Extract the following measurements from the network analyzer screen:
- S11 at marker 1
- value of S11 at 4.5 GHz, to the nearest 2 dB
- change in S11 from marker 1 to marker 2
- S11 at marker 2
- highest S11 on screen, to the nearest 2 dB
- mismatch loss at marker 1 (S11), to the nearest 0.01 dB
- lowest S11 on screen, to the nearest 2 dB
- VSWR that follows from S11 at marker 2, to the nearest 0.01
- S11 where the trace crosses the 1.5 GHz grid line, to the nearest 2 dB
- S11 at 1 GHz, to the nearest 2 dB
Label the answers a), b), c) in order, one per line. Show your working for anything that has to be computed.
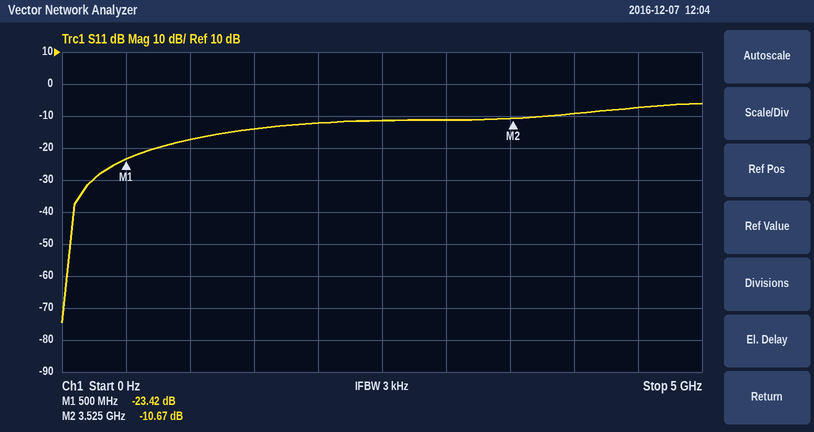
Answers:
a) -23.42 dB
b) -8 dB
c) -10.67 − (-23.42) = 12.75 dB
d) -10.67 dB
e) -6 dB
f) −10 log10(1 − 10^(-23.42/10)) ≈ 0.02 dB
g) -74 dB
h) (1 + 0.2928)/(1 − 0.2928) ≈ 1.83
i) -14 dB
j) -18 dB
